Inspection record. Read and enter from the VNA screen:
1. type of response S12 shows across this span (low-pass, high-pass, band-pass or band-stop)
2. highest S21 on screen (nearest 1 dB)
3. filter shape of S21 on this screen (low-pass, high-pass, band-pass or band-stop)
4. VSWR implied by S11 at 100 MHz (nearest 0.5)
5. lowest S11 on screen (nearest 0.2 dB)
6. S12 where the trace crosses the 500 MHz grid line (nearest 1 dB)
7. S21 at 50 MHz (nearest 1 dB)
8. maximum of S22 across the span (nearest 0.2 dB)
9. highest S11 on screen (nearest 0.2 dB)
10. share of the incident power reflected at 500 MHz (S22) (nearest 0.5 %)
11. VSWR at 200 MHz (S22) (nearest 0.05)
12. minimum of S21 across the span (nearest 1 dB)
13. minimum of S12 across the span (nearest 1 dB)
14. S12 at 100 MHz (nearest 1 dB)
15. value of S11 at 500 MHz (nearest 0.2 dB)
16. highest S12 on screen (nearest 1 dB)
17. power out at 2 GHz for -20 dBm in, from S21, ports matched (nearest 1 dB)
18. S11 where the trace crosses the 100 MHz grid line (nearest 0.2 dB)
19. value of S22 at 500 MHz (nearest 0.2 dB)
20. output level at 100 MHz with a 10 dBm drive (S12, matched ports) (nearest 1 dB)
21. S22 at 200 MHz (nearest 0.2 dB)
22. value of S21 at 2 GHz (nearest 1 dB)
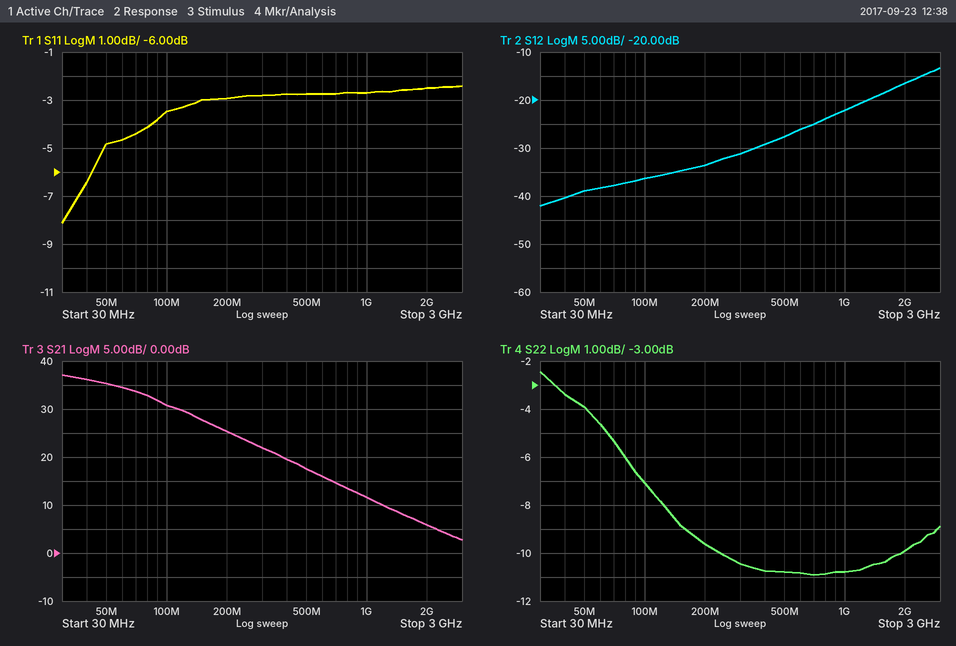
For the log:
high-pass
37 dB
low-pass
5.0
-8.2 dB
-28 dB
35 dB
-2.4 dB
-2.4 dB
8.5 %
2.00
3 dB
-42 dB
-36 dB
-2.8 dB
-13 dB
-14 dBm
-3.4 dB
-10.8 dB
-26 dBm
-9.6 dB
6 dB
